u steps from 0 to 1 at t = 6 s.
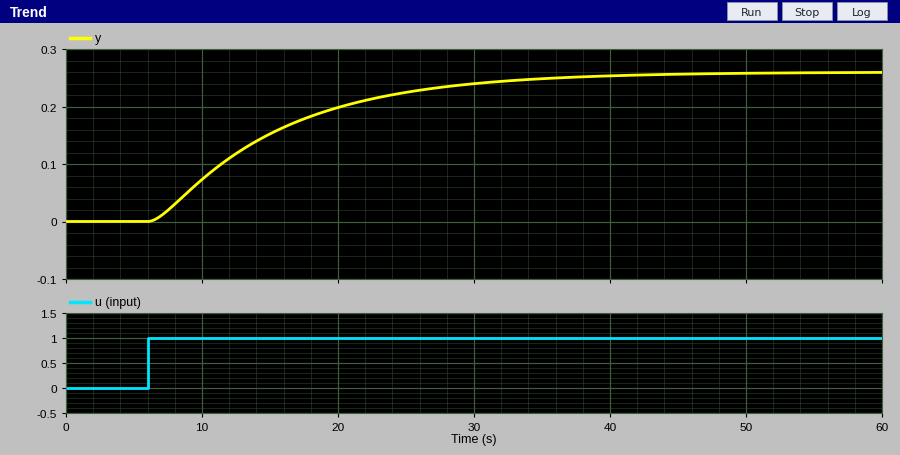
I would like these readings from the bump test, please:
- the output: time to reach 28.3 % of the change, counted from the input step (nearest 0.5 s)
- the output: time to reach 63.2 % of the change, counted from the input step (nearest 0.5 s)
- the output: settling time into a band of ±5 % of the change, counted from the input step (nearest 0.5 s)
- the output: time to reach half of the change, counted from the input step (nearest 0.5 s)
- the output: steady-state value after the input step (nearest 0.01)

4.0 s
10.0 s
28.0 s
7.5 s
0.26
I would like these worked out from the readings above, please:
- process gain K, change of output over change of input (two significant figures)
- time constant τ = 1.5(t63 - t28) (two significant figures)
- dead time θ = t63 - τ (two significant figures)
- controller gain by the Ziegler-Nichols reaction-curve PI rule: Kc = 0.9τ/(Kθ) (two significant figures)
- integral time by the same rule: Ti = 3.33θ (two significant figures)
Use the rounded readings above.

0.26
9.0 s
1.0 s
31
3.3 s
